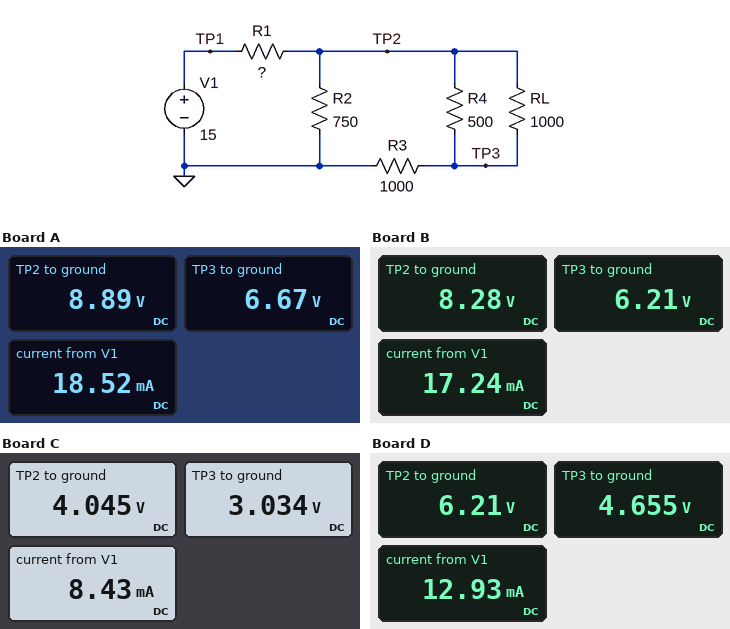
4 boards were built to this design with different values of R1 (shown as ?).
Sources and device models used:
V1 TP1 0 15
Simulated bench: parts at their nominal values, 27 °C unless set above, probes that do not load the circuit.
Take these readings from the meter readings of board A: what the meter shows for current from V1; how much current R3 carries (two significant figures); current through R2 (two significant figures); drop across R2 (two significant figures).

18.52 mA
6.7 mA
12 mA
8.9 V
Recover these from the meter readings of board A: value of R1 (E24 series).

330 Ω
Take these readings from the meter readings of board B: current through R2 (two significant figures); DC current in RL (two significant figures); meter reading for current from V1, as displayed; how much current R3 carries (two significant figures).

11 mA
2.1 mA
17.24 mA
6.2 mA
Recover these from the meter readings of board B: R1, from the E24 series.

390 Ω
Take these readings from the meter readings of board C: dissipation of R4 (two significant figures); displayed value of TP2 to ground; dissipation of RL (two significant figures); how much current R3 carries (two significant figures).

2.0 mW
4.045 V
1.0 mW
3.0 mA
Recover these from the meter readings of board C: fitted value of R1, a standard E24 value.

1.3 kΩ
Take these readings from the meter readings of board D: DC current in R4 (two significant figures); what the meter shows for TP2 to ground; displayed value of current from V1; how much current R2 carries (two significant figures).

3.1 mA
6.21 V
12.93 mA
8.3 mA
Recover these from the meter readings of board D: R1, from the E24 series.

680 Ω
